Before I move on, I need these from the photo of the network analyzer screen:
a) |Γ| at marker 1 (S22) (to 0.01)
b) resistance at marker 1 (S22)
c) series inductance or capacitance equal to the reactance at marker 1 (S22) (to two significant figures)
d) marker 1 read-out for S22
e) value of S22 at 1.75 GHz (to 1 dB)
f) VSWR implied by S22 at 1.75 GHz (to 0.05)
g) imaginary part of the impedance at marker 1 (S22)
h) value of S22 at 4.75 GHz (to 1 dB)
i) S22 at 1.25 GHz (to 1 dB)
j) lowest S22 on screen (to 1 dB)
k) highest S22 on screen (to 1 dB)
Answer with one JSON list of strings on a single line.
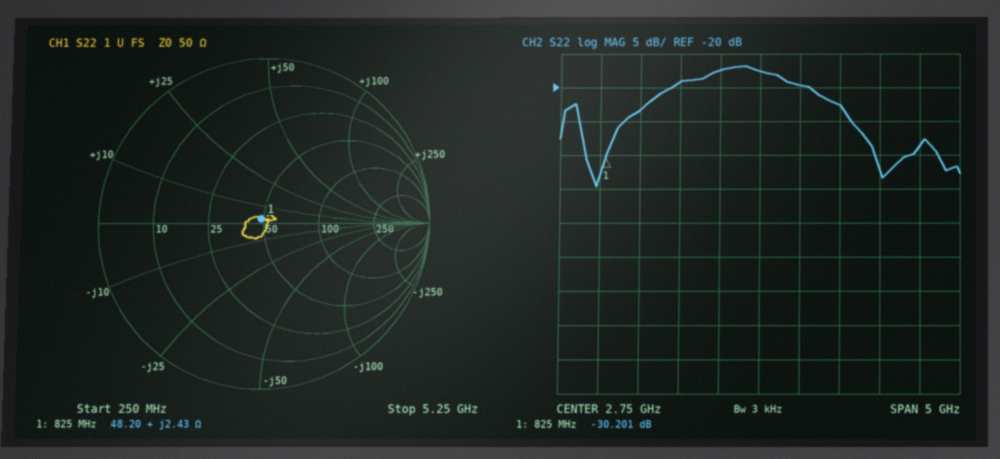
["0.03", "48.20 Ω", "470 pH", "-30.201 dB", "-19 dB", "1.25", "+2.43 Ω", "-29 dB", "-23 dB", "-35 dB", "-17 dB"]
